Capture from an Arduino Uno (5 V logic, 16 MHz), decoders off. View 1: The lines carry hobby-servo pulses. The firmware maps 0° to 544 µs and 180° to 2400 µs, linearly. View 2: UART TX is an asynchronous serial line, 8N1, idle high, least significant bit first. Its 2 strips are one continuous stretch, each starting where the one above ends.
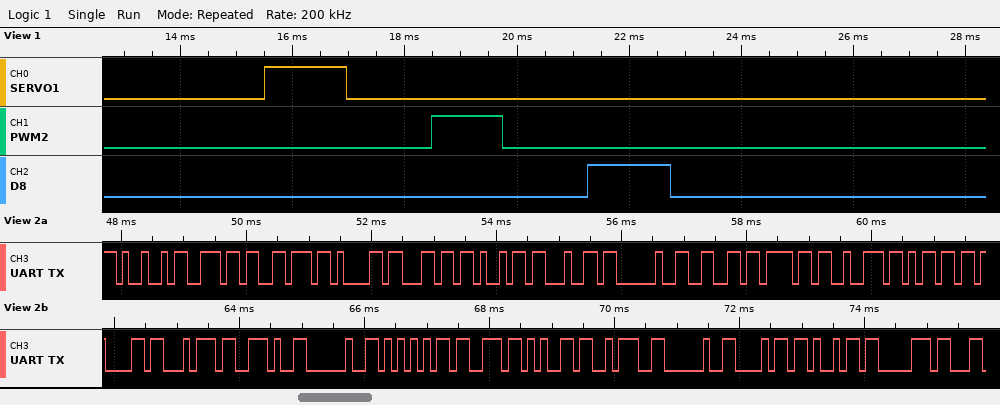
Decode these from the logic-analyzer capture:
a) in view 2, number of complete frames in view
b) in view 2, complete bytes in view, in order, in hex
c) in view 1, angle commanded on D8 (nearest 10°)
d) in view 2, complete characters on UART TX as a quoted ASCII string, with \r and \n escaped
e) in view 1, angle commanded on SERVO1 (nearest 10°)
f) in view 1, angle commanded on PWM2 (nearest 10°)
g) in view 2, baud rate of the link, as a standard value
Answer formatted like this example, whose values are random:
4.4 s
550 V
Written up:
24
49 6E 76 61 6C 69 64 20 66 6F 72 6D 61 74 2E 20 55 73 65 3A 20 68 69 70
90°
"Invalid format. Use: hip"
90°
70°
9600 baud
